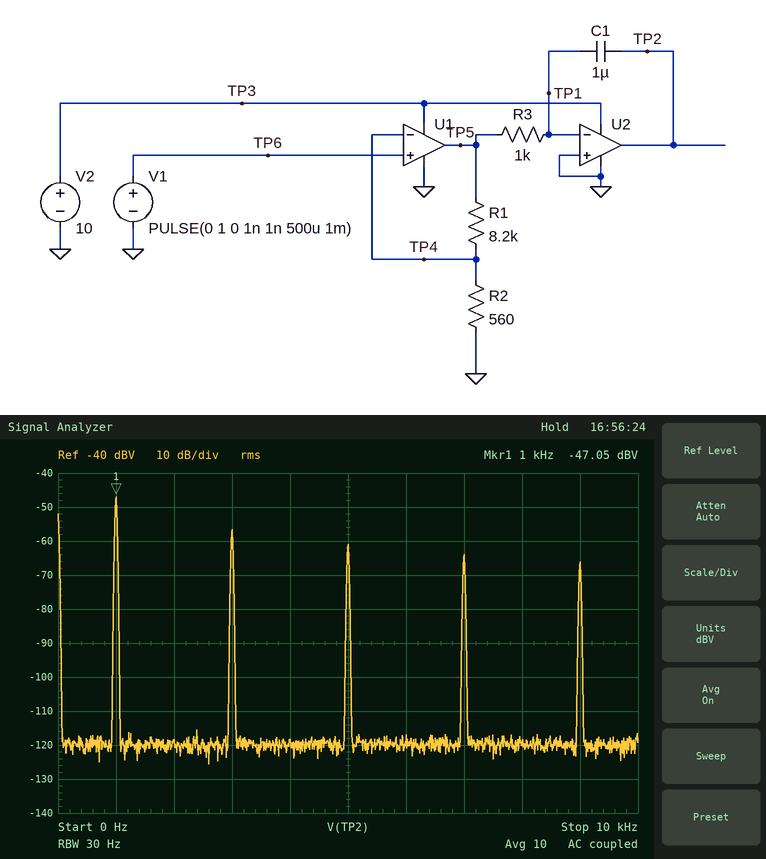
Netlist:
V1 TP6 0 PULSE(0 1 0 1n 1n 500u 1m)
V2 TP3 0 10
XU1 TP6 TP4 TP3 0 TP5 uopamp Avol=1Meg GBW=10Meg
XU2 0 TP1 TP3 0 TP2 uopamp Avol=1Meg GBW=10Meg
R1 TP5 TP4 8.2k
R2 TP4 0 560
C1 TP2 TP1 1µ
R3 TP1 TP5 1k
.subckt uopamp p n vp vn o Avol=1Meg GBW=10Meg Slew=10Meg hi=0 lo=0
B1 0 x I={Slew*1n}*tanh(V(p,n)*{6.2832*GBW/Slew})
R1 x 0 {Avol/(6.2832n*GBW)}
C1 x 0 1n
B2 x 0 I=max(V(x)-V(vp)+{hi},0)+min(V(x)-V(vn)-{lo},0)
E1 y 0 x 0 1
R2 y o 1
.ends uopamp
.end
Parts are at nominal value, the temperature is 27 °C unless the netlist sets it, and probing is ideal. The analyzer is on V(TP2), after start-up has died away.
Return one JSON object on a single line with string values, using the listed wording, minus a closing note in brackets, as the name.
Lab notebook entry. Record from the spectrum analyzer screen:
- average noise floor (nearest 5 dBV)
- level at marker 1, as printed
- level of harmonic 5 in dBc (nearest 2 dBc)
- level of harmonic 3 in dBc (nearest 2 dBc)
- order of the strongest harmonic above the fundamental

{"average noise floor": "-120 dBV", "level at marker 1, as printed": "-47.05 dBV", "level of harmonic 5 in dBc": "-14 dBc", "level of harmonic 3 in dBc": "-10 dBc", "order of the strongest harmonic above the fundamental": "3"}
